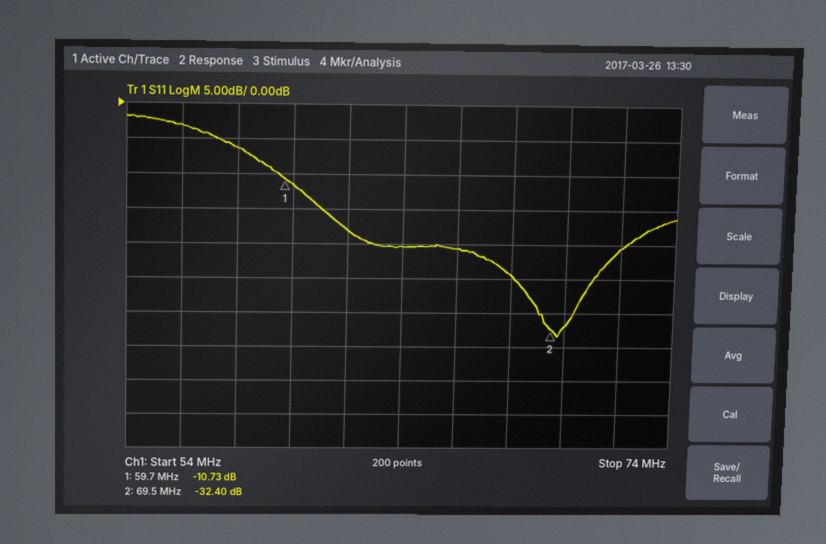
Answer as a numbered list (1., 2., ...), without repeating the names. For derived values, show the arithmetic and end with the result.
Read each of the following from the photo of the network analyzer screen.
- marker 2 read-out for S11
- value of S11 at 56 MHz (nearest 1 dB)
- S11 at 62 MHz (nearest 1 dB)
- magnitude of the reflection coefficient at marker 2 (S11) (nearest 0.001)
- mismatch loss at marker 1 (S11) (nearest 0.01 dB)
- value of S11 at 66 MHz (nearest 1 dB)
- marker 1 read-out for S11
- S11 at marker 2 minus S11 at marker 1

1. -32.40 dB
2. -3 dB
3. -18 dB
4. 10^(-32.4/20) ≈ 0.024
5. −10 log10(1 − 10^(-10.73/10)) ≈ 0.38 dB
6. -21 dB
7. -10.73 dB
8. -32.4 − (-10.73) = -21.67 dB
